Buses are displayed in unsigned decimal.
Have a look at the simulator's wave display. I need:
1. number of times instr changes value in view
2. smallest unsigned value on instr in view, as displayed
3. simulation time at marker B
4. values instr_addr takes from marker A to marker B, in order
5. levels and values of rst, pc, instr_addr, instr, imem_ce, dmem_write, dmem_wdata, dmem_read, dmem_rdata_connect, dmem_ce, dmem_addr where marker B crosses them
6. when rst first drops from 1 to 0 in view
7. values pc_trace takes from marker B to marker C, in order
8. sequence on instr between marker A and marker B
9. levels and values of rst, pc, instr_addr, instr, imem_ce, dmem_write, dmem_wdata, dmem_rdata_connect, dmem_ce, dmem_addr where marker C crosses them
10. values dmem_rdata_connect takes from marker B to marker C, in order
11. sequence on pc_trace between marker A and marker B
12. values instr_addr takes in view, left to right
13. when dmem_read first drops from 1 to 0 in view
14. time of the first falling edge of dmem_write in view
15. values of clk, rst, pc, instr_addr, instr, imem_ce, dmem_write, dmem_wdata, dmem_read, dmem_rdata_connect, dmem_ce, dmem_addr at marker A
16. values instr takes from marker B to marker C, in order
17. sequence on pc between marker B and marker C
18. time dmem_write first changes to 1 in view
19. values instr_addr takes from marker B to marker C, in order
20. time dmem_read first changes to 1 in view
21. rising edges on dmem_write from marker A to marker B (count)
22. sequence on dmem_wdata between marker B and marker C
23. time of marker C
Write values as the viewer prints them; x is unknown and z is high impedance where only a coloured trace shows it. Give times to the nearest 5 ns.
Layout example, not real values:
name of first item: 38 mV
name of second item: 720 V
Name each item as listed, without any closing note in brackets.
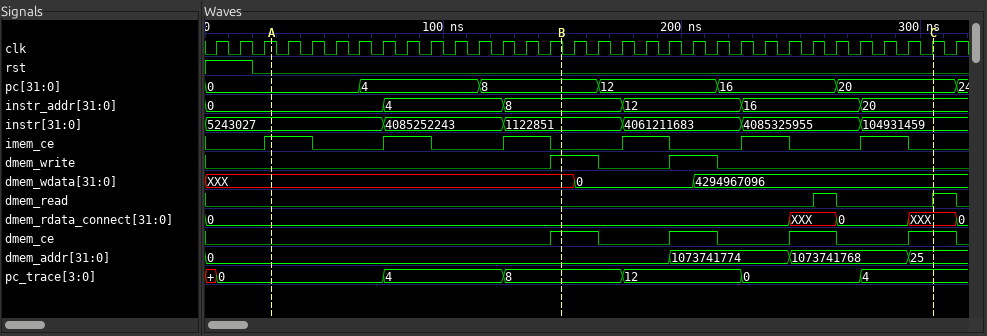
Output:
number of times instr changes value in view: 5
smallest unsigned value on instr in view, as displayed: 1122851
simulation time at marker B: 150 ns
values instr_addr takes from marker A to marker B, in order: 0, 4, 8
levels and values of rst, pc, instr_addr, instr, imem_ce, dmem_write, dmem_wdata, dmem_read, dmem_rdata_connect, dmem_ce, dmem_addr where marker B crosses them: rst=0, pc=8, instr_addr=8, instr=1122851, imem_ce=0, dmem_write=1, dmem_wdata=XXX, dmem_read=0, dmem_rdata_connect=0, dmem_ce=1, dmem_addr=0
when rst first drops from 1 to 0 in view: 20 ns
values pc_trace takes from marker B to marker C, in order: 8, 12, 0, 4
sequence on instr between marker A and marker B: 5243027, 4085252243, 1122851
levels and values of rst, pc, instr_addr, instr, imem_ce, dmem_write, dmem_wdata, dmem_rdata_connect, dmem_ce, dmem_addr where marker C crosses them: rst=0, pc=20, instr_addr=20, instr=104931459, imem_ce=0, dmem_write=0, dmem_wdata=4294967096, dmem_rdata_connect=XXX, dmem_ce=1, dmem_addr=25
values dmem_rdata_connect takes from marker B to marker C, in order: 0, XXX, 0, XXX
sequence on pc_trace between marker A and marker B: 0, 4, 8
values instr_addr takes in view, left to right: 0, 4, 8, 12, 16, 20
when dmem_read first drops from 1 to 0 in view: 265 ns
time of the first falling edge of dmem_write in view: 165 ns
values of clk, rst, pc, instr_addr, instr, imem_ce, dmem_write, dmem_wdata, dmem_read, dmem_rdata_connect, dmem_ce, dmem_addr at marker A: clk=1, rst=0, pc=0, instr_addr=0, instr=5243027, imem_ce=1, dmem_write=0, dmem_wdata=XXX, dmem_read=0, dmem_rdata_connect=0, dmem_ce=0, dmem_addr=0
values instr takes from marker B to marker C, in order: 1122851, 4061211683, 4085325955, 104931459
sequence on pc between marker B and marker C: 8, 12, 16, 20
time dmem_write first changes to 1 in view: 145 ns
values instr_addr takes from marker B to marker C, in order: 8, 12, 16, 20
time dmem_read first changes to 1 in view: 255 ns
rising edges on dmem_write from marker A to marker B: 1
sequence on dmem_wdata between marker B and marker C: XXX, 0, 4294967096
time of marker C: 305 ns
